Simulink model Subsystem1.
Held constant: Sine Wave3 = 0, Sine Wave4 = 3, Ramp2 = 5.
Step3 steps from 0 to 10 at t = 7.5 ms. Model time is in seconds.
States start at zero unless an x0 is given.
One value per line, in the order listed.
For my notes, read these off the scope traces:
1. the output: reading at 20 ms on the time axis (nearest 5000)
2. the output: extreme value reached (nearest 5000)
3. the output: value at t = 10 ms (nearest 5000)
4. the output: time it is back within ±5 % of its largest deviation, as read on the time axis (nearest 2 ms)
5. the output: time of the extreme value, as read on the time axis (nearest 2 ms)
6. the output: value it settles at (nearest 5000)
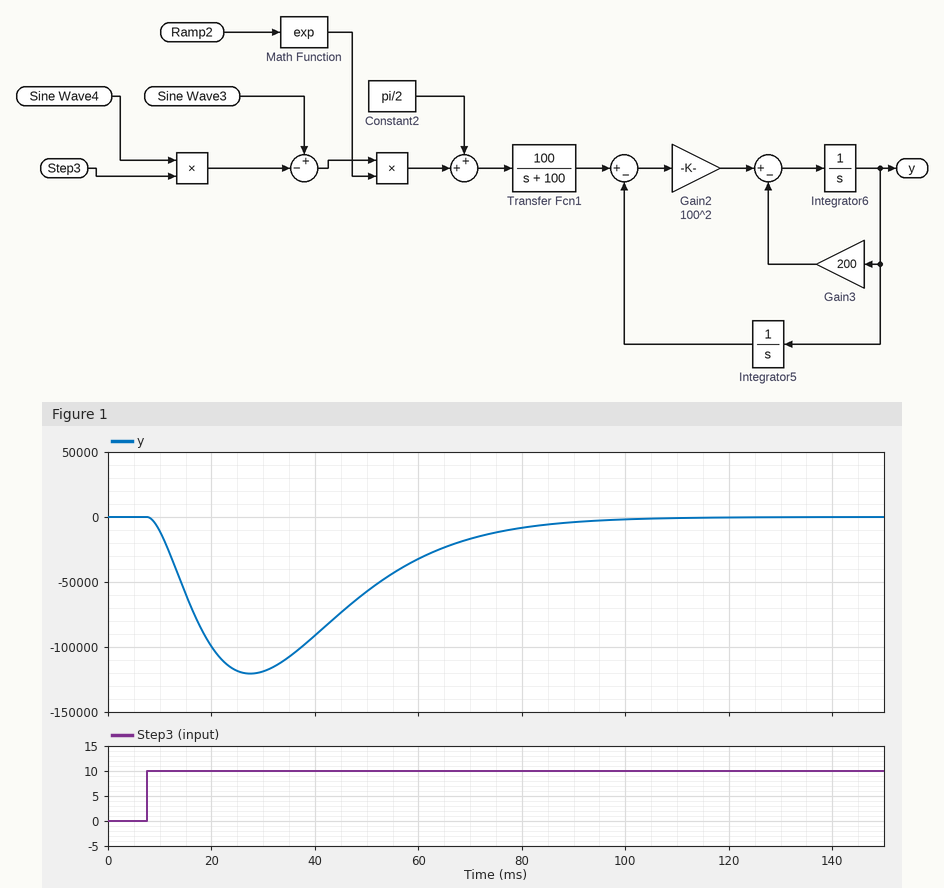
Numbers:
-100000
-120000
-10000
84 ms
28 ms
0
